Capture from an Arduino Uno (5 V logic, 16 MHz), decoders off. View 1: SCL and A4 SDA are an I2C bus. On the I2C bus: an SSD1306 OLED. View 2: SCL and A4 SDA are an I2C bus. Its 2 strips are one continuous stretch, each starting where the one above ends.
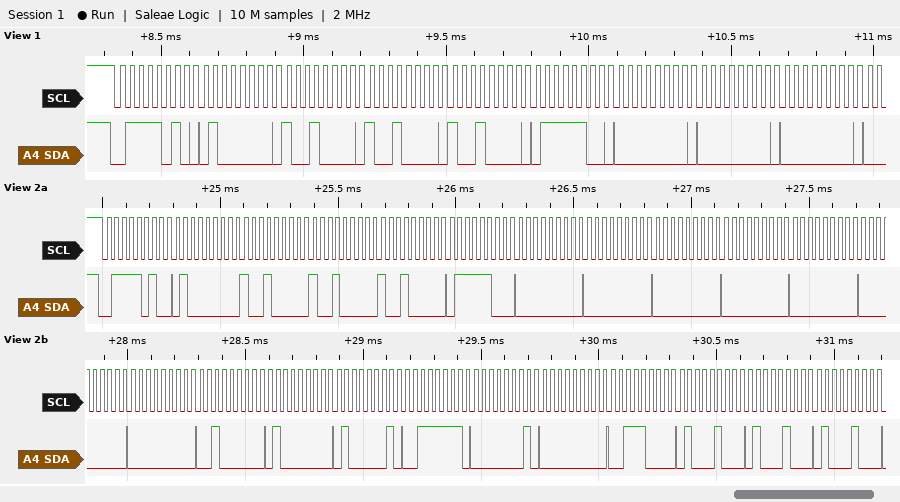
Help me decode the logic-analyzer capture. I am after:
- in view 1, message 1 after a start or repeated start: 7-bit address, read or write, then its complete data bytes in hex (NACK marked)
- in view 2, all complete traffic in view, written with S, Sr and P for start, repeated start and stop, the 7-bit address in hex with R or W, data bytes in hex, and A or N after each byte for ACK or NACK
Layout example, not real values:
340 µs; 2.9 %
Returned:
0x3D write: 40 90 90 90 7C 00 00 00; S 3DW A 40 A 90 A 90 A 90 A 7C A 00 A 00 A 00 A 00 A 00 A 00 A 00 A 20 A 40 A 41 A 3F A 01 A 00 A 38 A 44 A 44 A 44 A
